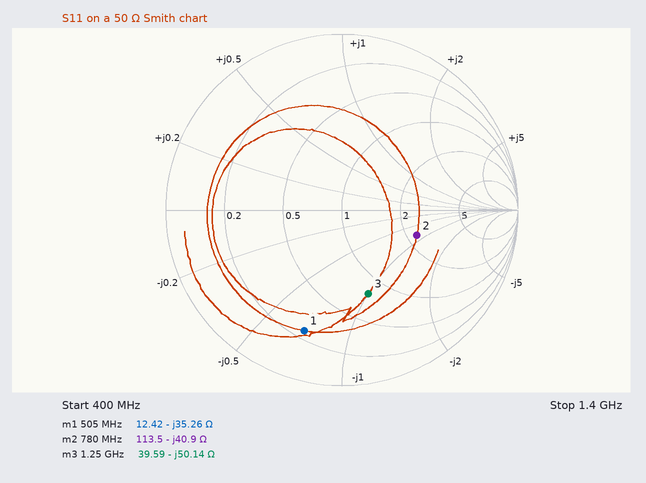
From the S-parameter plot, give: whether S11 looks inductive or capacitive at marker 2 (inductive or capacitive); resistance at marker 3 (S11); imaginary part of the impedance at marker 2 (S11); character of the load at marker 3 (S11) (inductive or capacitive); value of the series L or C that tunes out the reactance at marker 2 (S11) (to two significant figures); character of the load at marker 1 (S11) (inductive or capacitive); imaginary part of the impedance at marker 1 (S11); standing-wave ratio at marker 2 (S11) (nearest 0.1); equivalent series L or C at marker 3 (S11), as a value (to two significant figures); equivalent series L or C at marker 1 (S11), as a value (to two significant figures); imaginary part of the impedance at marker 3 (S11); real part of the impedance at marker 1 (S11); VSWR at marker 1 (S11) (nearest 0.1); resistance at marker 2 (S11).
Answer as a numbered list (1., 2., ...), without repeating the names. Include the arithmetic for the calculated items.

1. capacitive
2. 39.59 Ω
3. -40.9 Ω
4. capacitive
5. L = 40.9 Ω/(2π × 780 MHz) ≈ 8.3 nH
6. capacitive
7. -35.26 Ω
8. 2.6
9. C = 1/(2π × 1.25 GHz × 50.14 Ω) ≈ 2.5 pF
10. C = 1/(2π × 505 MHz × 35.26 Ω) ≈ 8.9 pF
11. -50.14 Ω
12. 12.42 Ω
13. 6.1
14. 113.5 Ω
